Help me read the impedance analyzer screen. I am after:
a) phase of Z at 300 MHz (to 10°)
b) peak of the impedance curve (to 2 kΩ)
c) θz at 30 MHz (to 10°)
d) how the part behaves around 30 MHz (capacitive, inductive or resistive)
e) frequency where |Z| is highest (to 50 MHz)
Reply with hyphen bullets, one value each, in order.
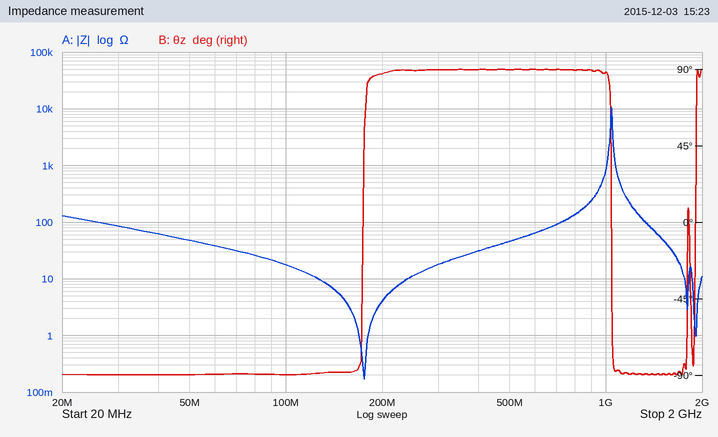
- 90°
- 10 kΩ
- -90°
- capacitive
- 1.05 GHz
